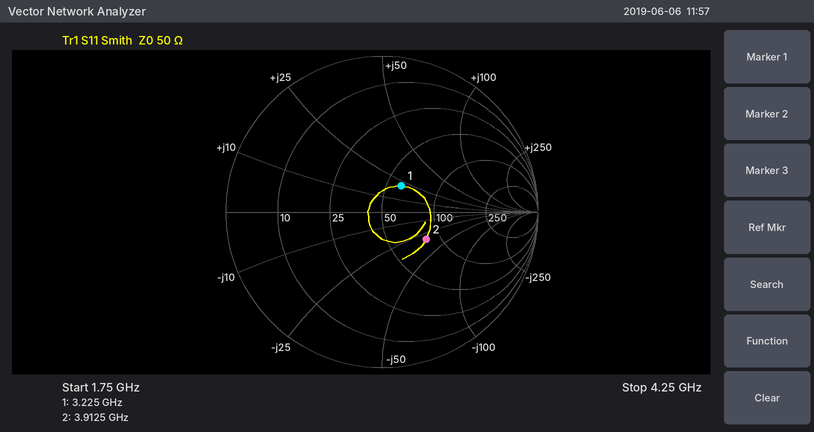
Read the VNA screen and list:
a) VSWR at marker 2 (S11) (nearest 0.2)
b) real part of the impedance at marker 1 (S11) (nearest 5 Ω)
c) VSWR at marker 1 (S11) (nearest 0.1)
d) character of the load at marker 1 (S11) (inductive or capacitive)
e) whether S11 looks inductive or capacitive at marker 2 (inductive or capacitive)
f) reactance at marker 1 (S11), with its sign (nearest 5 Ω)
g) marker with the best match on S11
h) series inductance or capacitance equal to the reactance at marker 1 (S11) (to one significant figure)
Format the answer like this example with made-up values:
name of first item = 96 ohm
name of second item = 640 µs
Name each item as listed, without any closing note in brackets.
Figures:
VSWR at marker 2 (S11) = 2.0
real part of the impedance at marker 1 (S11) = 60 Ω
VSWR at marker 1 (S11) = 1.5
character of the load at marker 1 (S11) = inductive
whether S11 looks inductive or capacitive at marker 2 = capacitive
reactance at marker 1 (S11), with its sign = +20 Ω
marker with the best match on S11 = marker 1
series inductance or capacitance equal to the reactance at marker 1 (S11) = 1 nH
